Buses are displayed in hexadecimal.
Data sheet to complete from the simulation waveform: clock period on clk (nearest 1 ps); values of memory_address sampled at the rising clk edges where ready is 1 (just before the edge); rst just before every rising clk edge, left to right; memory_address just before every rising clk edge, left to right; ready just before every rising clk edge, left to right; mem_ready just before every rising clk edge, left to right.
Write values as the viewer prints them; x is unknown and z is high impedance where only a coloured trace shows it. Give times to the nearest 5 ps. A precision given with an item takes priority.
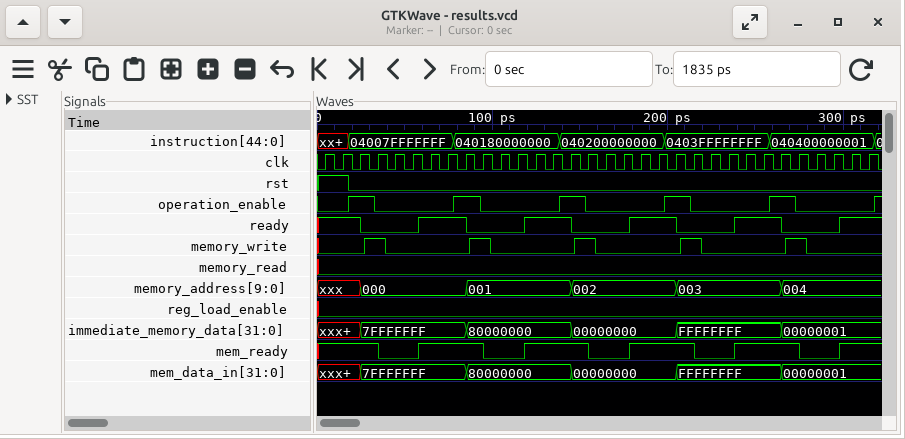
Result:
10 ps
xxx, xxx, xxx, 000, 000, 000, 001, 001, 001, 002, 002, 002, 003, 003, 003, 004, 004
1 1 0 0 0 0 0 0 0 0 0 0 0 0 0 0 0 0 0 0 0 0 0 0 0 0 0 0 0 0 0 0
xxx, xxx, xxx, 000, 000, 000, 000, 000, 000, 001, 001, 001, 001, 001, 001, 002, 002, 002, 002, 002, 002, 003, 003, 003, 003, 003, 003, 004, 004, 004, 004, 004
1 1 1 0 0 0 1 1 1 0 0 0 1 1 1 0 0 0 1 1 1 0 0 0 1 1 1 0 0 0 1 1
1 1 1 1 0 0 1 1 1 1 0 0 1 1 1 1 0 0 1 1 1 1 0 0 1 1 1 1 0 0 1 1
